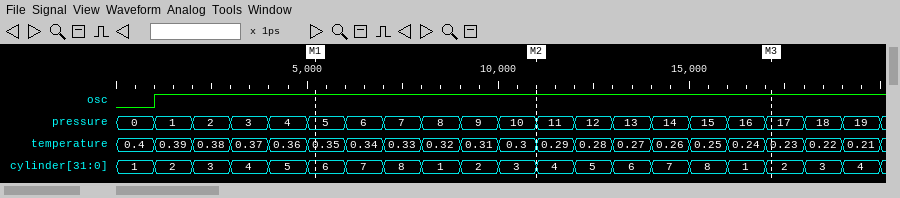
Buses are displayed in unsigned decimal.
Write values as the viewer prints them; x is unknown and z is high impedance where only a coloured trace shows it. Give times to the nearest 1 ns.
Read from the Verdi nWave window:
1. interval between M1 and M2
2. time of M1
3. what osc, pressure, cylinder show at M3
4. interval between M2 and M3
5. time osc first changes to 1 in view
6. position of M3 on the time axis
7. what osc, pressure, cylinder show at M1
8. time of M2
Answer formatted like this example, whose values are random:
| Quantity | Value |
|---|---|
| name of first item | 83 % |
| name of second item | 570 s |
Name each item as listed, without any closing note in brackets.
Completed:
| Quantity | Value |
|---|---|
| interval between M1 and M2 | 6 ns |
| time of M1 | 5 ns |
| what osc, pressure, cylinder show at M3 | osc=1, pressure=17, cylinder=2 |
| interval between M2 and M3 | 6 ns |
| time osc first changes to 1 in view | 1 ns |
| position of M3 on the time axis | 17 ns |
| what osc, pressure, cylinder show at M1 | osc=1, pressure=5, cylinder=6 |
| time of M2 | 11 ns |
